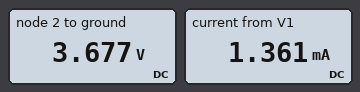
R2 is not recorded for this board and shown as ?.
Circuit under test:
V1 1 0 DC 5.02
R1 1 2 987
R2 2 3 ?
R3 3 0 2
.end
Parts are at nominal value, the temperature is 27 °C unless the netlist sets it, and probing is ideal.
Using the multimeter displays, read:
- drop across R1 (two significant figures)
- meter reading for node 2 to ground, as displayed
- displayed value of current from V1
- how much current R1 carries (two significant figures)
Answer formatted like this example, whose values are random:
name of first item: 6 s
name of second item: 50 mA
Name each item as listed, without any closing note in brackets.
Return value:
drop across R1: 1.3 V
meter reading for node 2 to ground, as displayed: 3.677 V
displayed value of current from V1: 1.361 mA
how much current R1 carries: 1.4 mA
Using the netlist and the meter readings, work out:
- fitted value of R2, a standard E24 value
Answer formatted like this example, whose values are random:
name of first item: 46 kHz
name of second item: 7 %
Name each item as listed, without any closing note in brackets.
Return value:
fitted value of R2, a standard E24 value: 2.7 kΩ
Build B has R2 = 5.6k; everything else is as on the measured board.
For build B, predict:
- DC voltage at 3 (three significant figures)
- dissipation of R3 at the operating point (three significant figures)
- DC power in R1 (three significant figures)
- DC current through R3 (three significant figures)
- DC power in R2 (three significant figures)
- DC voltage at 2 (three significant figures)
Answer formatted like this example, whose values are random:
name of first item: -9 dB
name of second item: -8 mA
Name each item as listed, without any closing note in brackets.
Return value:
DC voltage at 3: 1.52 mV
dissipation of R3 at the operating point: 1.16 µW
DC power in R1: 573 µW
DC current through R3: 762 µA
DC power in R2: 3.25 mW
DC voltage at 2: 4.27 V
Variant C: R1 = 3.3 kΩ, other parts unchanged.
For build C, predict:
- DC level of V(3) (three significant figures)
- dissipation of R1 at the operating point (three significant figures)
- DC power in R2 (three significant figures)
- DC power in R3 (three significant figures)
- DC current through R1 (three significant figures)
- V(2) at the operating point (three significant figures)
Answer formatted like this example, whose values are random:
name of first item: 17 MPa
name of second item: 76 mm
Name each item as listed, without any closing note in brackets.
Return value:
DC level of V(3): 1.67 mV
dissipation of R1 at the operating point: 2.31 mW
DC power in R2: 1.89 mW
DC power in R3: 1.40 µW
DC current through R1: 836 µA
V(2) at the operating point: 2.26 V
